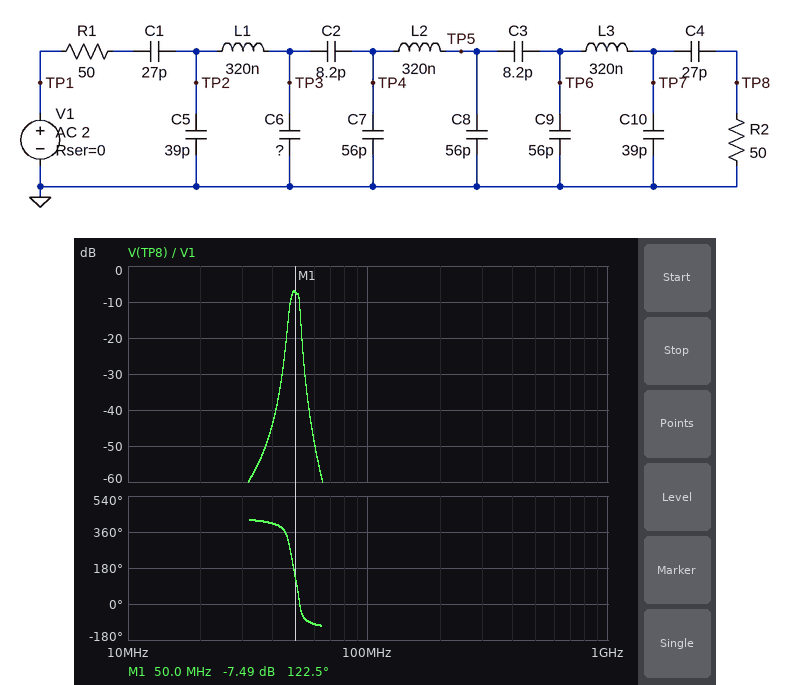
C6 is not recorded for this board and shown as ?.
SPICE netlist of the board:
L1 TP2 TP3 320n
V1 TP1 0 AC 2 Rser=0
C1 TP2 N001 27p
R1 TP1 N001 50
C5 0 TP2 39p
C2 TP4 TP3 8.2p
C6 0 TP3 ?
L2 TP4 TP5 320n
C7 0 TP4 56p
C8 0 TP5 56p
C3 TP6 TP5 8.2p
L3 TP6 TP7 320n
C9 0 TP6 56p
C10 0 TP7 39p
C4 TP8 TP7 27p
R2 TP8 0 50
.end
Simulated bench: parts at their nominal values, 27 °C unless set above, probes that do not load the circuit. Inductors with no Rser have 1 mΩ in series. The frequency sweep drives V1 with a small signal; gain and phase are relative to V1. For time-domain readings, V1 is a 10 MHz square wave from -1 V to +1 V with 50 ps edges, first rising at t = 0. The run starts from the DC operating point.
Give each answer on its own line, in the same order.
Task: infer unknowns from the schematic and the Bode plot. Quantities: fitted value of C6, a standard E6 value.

68 pF
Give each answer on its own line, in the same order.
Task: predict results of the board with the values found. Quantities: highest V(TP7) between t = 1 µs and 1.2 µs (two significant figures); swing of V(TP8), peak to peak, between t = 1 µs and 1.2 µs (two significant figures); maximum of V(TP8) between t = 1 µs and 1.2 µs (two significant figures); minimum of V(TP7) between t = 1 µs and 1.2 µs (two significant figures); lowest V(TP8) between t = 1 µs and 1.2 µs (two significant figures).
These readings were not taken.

280 mV
220 mV
110 mV
-280 mV
-110 mV
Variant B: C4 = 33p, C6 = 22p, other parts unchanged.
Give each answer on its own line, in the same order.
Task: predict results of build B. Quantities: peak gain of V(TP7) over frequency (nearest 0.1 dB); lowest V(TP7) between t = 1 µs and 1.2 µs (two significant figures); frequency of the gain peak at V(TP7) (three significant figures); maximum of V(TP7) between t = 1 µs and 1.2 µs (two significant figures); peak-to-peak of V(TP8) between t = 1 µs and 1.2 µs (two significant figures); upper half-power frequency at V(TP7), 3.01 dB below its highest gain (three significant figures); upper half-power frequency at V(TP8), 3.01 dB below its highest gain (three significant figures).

-3.8 dB
-170 mV
50.0 MHz
170 mV
150 mV
51.0 MHz
51.1 MHz
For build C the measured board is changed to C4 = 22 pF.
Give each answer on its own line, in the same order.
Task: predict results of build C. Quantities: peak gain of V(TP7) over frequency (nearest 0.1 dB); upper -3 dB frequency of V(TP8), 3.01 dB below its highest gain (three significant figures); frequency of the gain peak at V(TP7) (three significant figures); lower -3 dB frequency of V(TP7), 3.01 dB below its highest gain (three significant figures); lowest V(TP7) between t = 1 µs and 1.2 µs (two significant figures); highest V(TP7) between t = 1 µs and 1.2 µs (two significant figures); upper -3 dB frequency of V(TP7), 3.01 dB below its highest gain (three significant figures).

3.5 dB
51.1 MHz
49.4 MHz
48.1 MHz
-340 mV
340 mV
50.9 MHz
